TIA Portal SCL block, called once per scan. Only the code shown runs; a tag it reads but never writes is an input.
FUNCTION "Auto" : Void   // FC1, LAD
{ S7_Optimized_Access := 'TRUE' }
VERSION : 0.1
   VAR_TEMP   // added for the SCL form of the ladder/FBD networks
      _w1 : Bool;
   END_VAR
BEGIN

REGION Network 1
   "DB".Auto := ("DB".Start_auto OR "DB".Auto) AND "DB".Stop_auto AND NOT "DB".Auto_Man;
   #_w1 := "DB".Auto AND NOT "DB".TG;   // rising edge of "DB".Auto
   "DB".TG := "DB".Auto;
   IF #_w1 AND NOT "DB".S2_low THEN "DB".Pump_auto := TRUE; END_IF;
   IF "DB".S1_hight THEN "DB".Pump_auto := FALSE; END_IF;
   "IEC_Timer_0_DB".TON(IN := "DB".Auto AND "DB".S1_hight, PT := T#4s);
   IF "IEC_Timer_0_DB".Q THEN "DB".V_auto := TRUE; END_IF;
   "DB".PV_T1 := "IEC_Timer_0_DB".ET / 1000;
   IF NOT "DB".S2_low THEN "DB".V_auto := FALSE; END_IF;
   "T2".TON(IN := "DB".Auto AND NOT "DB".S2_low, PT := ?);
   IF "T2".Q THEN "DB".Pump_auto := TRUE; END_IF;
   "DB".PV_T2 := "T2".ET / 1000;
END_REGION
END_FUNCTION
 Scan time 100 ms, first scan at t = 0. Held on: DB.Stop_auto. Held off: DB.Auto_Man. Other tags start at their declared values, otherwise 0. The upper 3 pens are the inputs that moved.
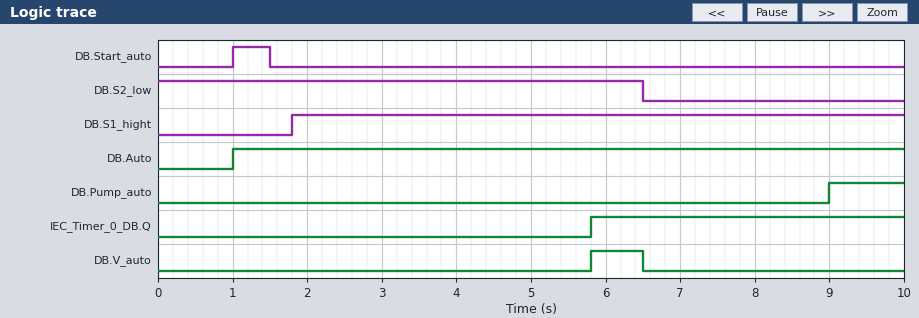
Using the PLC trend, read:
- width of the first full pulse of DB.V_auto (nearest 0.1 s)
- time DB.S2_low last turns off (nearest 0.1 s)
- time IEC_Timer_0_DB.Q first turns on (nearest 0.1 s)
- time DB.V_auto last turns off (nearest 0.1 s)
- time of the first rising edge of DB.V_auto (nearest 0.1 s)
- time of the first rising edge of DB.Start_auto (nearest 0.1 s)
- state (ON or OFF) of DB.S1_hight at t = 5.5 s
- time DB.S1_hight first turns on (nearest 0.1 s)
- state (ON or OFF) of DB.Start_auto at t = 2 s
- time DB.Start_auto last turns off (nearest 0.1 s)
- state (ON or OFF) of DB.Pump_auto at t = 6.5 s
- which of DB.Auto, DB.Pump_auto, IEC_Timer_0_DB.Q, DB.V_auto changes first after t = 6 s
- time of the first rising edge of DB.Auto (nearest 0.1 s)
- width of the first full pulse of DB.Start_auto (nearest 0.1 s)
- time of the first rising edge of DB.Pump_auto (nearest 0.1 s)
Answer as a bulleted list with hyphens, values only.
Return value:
- 0.7 s
- 6.5 s
- 5.8 s
- 6.5 s
- 5.8 s
- 1.0 s
- ON
- 1.8 s
- OFF
- 1.5 s
- OFF
- DB.V_auto
- 1.0 s
- 0.5 s
- 9.0 s
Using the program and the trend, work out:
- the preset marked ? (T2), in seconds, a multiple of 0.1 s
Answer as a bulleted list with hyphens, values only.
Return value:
- 2.5 s
